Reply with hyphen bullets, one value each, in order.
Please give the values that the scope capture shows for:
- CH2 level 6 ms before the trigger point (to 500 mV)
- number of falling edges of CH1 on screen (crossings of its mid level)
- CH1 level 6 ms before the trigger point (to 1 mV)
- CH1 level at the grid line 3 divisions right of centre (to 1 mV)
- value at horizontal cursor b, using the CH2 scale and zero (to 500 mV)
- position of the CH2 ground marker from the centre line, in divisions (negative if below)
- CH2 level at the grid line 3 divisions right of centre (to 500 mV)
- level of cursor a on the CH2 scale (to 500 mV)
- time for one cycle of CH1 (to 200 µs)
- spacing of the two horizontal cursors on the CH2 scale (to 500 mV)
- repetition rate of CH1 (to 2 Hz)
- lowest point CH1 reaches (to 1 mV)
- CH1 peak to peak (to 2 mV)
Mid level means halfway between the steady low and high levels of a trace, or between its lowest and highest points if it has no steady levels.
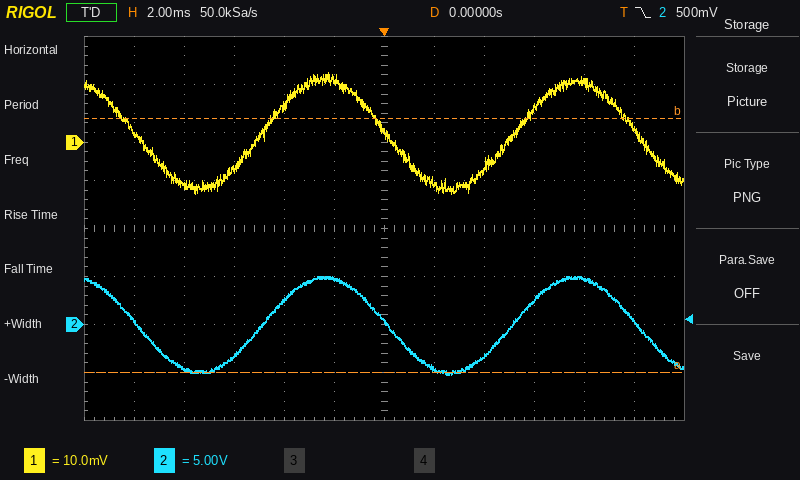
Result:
- -3.0 V
- 3
- -5 mV
- 7 mV
- 21.5 V
- -2.0 div
- 2.5 V
- -5.0 V
- 10.0 ms
- 26.5 V
- 100 Hz
- -11 mV
- 26 mV
